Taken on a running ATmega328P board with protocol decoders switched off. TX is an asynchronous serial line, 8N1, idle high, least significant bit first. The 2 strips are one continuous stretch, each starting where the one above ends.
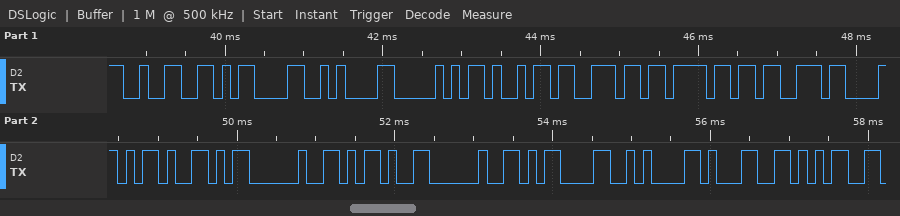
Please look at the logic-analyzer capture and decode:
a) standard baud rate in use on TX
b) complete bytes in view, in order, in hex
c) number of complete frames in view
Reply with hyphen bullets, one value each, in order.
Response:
- 9600 baud
- 32 0D 0A 50 69 6E 6F 73 58 59 20 2D 20 0D 0A 31 35
- 17
